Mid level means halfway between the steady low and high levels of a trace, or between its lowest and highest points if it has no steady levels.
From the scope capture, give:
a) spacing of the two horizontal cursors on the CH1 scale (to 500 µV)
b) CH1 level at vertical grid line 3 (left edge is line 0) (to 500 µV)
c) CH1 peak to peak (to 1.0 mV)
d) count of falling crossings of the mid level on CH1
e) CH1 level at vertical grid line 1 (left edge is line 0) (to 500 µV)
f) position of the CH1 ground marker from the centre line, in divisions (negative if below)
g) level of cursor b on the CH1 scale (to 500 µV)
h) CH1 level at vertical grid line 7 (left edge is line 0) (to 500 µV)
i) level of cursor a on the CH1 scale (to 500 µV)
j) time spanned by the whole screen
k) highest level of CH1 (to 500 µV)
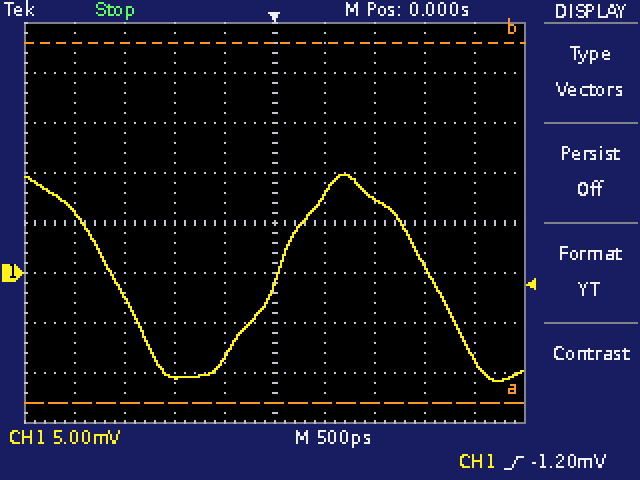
36.0 mV
-10.5 mV
21.0 mV
2
6.0 mV
-1.0 div
23.0 mV
7.5 mV
-13.0 mV
5 ns
10.0 mV
